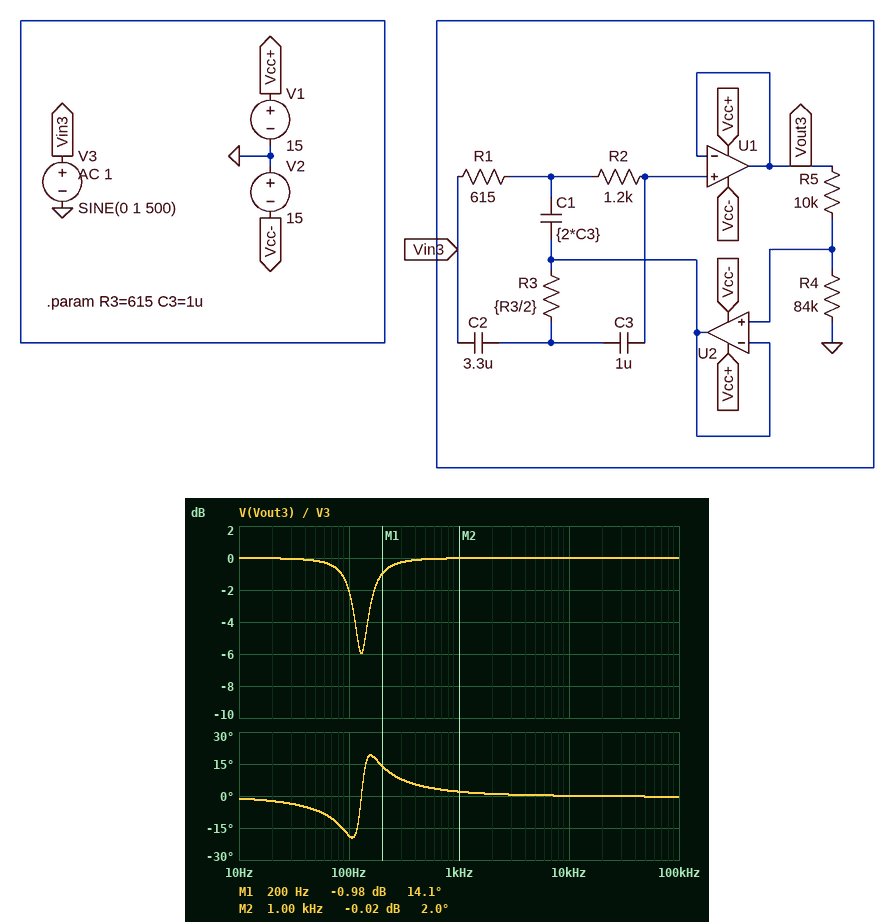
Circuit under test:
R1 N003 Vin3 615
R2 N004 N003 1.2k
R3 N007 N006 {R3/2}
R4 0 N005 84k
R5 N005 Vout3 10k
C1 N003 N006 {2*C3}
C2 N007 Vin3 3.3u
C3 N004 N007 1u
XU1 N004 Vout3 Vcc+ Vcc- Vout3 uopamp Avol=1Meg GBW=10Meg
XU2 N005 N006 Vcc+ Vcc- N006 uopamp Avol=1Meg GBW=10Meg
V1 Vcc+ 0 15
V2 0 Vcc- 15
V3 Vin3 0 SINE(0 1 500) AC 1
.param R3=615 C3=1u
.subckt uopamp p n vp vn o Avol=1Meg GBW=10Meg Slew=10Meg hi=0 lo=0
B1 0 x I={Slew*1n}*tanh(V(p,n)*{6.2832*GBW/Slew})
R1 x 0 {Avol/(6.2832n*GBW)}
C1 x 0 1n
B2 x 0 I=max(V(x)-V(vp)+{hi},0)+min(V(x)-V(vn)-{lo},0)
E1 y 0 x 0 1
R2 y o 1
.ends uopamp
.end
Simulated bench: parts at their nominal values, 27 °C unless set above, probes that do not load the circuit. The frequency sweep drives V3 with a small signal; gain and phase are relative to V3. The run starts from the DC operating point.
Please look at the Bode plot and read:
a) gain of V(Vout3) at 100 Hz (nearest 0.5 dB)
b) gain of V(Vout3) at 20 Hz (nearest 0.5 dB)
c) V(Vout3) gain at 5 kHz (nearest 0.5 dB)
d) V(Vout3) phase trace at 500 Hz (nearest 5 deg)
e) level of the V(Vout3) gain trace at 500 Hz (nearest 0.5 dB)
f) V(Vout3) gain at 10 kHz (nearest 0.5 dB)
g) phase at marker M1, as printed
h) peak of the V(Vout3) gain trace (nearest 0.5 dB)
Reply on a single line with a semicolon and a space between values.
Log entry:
-2.0 dB; 0 dB; 0 dB; 5 deg; 0 dB; 0 dB; 14.1 deg; 0 dB
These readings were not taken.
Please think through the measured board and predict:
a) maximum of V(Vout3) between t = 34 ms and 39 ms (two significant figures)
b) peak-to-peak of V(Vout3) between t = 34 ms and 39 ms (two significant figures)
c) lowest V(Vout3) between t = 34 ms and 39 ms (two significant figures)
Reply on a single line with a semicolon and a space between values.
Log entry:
990 mV; 2.0 V; -990 mV
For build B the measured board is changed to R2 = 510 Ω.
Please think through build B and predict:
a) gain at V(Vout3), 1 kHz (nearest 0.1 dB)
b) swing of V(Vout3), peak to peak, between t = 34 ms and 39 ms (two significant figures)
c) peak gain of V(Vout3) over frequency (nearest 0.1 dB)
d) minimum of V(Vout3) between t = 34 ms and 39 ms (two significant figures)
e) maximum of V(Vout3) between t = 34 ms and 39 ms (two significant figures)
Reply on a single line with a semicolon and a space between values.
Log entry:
-0.1 dB; 1.9 V; 0 dB; -960 mV; 960 mV
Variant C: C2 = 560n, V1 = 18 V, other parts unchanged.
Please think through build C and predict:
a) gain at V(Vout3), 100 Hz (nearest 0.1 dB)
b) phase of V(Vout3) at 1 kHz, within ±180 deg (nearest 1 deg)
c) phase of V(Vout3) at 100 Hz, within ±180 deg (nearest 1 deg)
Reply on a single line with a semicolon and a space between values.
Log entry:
0 dB; 8 deg; -14 deg
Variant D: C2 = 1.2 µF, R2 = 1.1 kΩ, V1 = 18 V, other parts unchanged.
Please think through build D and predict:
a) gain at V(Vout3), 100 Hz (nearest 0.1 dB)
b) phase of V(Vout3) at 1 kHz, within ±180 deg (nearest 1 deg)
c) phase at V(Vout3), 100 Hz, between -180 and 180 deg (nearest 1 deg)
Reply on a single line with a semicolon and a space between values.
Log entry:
-0.2 dB; 4 deg; -15 deg
